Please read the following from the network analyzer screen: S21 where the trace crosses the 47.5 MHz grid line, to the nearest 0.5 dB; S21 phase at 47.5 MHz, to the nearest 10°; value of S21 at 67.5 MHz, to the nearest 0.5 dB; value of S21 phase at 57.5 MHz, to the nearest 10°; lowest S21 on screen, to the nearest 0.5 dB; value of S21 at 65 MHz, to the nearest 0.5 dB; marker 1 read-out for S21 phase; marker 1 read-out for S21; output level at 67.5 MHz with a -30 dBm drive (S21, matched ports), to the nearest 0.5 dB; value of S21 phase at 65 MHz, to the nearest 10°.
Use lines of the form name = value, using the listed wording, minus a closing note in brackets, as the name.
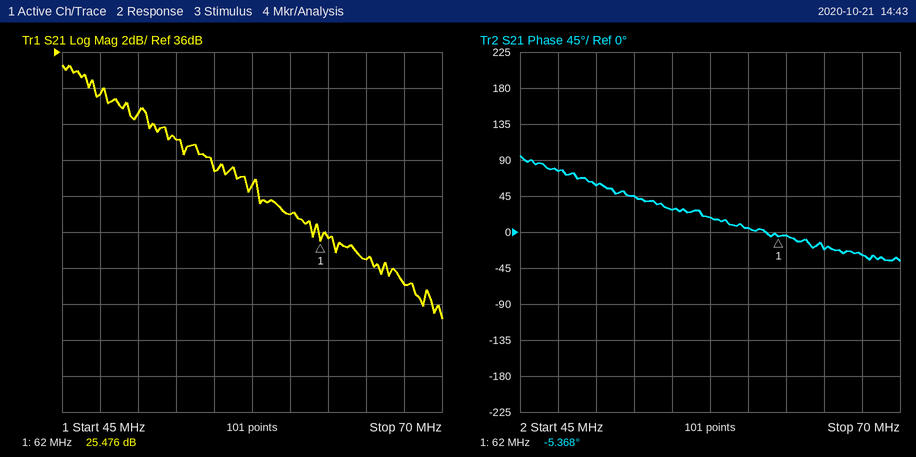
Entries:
S21 where the trace crosses the 47.5 MHz grid line, to the nearest 0.5 dB = 33.5 dB
S21 phase at 47.5 MHz, to the nearest 10° = 80°
value of S21 at 67.5 MHz, to the nearest 0.5 dB = 23.0 dB
value of S21 phase at 57.5 MHz, to the nearest 10° = 20°
lowest S21 on screen, to the nearest 0.5 dB = 21.0 dB
value of S21 at 65 MHz, to the nearest 0.5 dB = 24.5 dB
marker 1 read-out for S21 phase = -5.368°
marker 1 read-out for S21 = 25.476 dB
output level at 67.5 MHz with a -30 dBm drive (S21, matched ports), to the nearest 0.5 dB = -7.0 dBm
value of S21 phase at 65 MHz, to the nearest 10° = -20°
